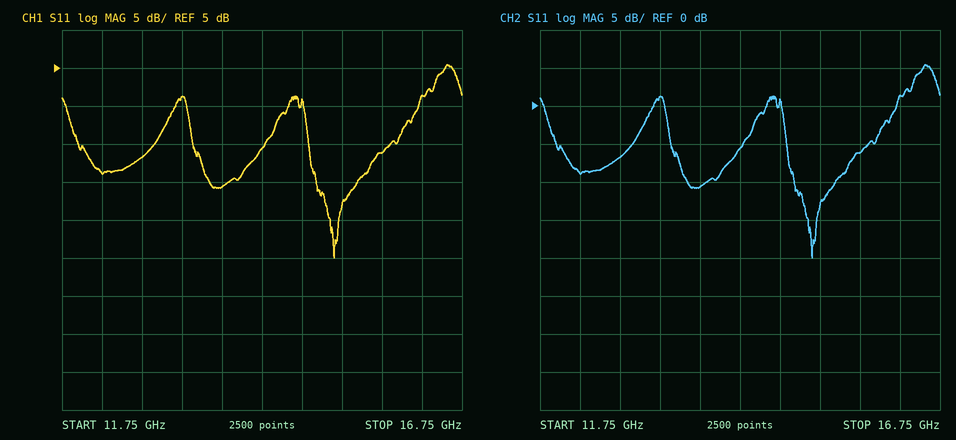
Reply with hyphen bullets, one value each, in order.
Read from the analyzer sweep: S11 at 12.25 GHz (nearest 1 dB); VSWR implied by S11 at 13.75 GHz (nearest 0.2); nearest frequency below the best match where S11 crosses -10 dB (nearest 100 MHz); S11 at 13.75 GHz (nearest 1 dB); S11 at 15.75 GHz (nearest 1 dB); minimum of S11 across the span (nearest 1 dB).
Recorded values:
- -9 dB
- 1.8
- 14.9 GHz
- -11 dB
- -6 dB
- -20 dB
